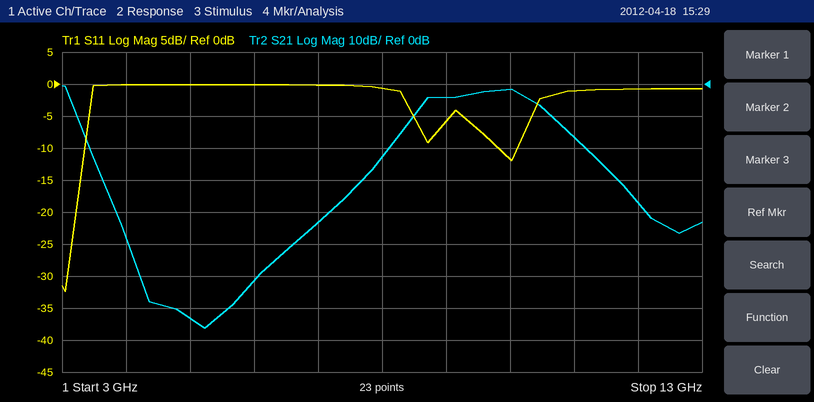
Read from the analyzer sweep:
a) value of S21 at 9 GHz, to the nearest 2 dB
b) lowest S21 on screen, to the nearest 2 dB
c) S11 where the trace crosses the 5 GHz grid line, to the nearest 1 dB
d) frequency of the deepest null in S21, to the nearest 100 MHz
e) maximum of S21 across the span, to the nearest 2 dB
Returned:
-4 dB
-76 dB
0 dB
5.2 GHz
0 dB
